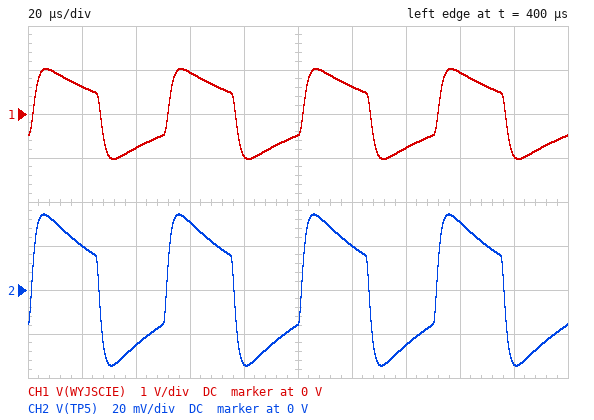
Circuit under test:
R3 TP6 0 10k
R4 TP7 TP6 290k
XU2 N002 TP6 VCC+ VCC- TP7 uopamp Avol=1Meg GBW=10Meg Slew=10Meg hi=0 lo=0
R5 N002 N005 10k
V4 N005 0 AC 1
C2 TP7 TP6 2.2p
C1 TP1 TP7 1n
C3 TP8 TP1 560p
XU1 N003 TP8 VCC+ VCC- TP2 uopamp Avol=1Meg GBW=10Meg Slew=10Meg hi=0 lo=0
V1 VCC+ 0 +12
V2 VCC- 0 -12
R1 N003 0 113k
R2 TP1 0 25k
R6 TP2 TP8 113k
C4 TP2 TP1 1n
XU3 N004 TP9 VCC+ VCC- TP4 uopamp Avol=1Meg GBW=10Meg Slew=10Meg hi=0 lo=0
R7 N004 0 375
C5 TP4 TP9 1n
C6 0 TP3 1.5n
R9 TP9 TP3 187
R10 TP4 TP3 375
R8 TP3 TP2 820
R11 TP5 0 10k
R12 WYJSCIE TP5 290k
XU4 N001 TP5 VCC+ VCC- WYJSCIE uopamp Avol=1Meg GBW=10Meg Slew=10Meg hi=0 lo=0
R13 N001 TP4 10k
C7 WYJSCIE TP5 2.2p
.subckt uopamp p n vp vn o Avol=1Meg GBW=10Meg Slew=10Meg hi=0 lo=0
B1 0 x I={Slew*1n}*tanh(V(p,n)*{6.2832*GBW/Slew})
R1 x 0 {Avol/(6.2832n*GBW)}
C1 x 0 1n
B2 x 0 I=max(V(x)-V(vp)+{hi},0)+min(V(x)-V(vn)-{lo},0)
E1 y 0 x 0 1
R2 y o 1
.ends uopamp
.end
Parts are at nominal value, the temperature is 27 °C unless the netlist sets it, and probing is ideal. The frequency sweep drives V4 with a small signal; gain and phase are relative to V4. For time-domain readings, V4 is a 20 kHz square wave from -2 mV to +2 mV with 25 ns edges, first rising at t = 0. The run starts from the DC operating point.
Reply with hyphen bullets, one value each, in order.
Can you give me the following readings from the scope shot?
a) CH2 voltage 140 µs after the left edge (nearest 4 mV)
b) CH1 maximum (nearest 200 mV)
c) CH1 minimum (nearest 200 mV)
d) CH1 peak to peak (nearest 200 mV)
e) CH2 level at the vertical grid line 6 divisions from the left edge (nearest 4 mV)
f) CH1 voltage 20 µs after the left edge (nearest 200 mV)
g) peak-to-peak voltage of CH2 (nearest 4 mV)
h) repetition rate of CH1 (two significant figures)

- -24 mV
- 1.0 V
- -1.0 V
- 2.0 V
- 20 mV
- 600 mV
- 68 mV
- 20 kHz
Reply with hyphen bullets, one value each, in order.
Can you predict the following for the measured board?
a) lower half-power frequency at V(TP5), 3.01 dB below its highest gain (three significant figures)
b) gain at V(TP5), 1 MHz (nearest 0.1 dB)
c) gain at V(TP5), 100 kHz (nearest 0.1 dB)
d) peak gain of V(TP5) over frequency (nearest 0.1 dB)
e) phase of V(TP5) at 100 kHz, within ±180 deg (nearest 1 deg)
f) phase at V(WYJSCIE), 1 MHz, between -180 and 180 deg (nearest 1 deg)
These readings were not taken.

- 4.46 kHz
- -13.6 dB
- 19.6 dB
- 22.5 dB
- -69 deg
- 58 deg
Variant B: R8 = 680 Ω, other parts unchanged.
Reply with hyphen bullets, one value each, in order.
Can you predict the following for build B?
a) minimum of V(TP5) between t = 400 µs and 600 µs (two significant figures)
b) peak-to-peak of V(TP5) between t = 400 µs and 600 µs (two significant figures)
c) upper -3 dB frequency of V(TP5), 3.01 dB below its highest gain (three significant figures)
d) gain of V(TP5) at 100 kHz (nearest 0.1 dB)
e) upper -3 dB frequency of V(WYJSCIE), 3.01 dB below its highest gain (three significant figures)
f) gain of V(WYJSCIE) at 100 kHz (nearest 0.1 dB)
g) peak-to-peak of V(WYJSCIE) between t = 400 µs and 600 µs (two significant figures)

- -41 mV
- 83 mV
- 102 kHz
- 21.2 dB
- 91.8 kHz
- 50.1 dB
- 2.5 V
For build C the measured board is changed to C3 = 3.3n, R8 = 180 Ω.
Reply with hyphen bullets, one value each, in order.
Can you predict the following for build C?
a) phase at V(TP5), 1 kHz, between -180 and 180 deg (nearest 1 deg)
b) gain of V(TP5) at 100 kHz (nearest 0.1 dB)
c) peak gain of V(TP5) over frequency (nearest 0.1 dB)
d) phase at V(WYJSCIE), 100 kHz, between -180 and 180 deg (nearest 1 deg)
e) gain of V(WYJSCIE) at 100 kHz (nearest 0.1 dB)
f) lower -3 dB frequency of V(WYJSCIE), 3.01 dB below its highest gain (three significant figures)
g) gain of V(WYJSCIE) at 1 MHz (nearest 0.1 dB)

- 126 deg
- 32.0 dB
- 35.9 dB
- -102 deg
- 60.9 dB
- 1.60 kHz
- 14.5 dB
